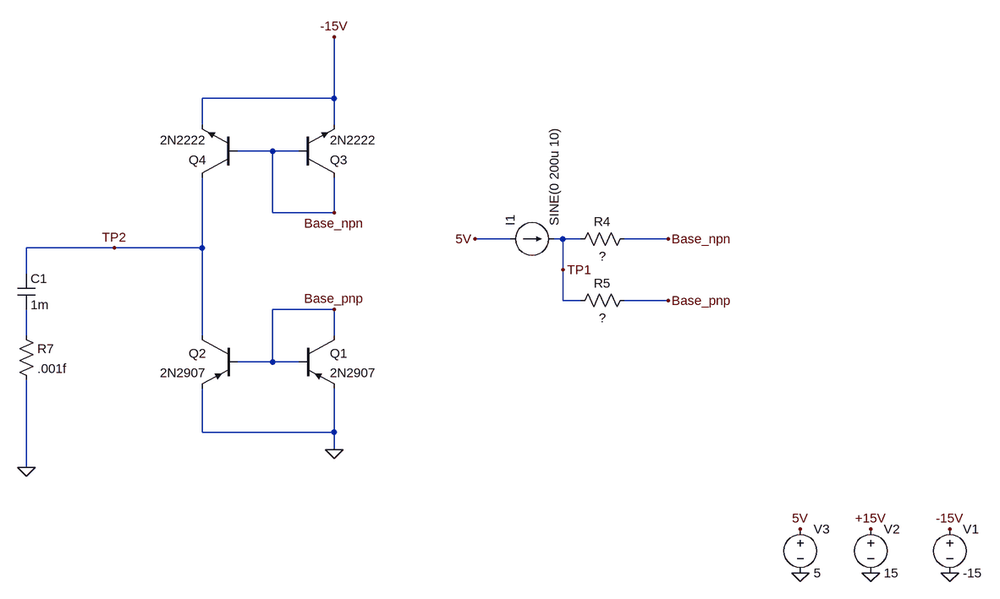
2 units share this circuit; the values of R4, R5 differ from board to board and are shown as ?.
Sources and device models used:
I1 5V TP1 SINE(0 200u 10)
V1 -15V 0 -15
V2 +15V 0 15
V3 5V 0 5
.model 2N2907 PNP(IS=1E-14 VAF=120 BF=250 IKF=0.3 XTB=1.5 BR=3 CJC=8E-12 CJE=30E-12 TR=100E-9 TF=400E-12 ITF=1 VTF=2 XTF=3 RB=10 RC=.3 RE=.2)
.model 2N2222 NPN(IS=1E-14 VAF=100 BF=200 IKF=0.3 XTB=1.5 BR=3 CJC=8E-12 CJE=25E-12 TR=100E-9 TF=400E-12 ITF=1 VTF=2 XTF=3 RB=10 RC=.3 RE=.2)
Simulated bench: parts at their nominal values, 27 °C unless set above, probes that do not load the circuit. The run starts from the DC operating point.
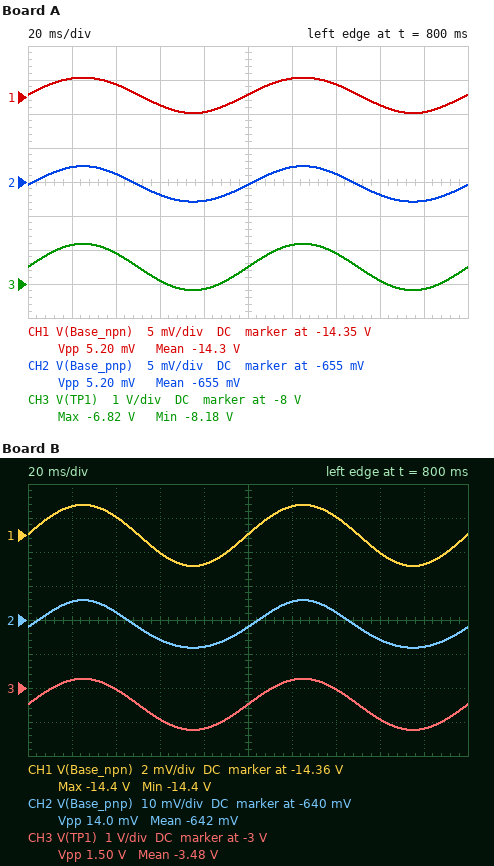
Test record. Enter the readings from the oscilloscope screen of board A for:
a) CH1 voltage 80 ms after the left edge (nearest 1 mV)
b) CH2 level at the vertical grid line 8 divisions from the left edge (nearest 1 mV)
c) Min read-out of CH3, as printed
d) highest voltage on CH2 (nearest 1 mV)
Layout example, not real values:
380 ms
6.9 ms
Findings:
-14.347 V
-657 mV
-8.18 V
-653 mV
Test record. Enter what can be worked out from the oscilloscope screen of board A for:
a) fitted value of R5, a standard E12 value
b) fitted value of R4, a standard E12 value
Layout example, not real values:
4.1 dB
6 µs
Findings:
6.8 kΩ
6.8 kΩ
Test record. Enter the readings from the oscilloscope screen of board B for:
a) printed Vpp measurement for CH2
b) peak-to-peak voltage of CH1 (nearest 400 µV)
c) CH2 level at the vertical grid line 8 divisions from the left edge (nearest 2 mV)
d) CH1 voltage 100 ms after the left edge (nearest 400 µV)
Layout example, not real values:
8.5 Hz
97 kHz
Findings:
14.0 mV
3.6 mV
-646 mV
-14.3580 V
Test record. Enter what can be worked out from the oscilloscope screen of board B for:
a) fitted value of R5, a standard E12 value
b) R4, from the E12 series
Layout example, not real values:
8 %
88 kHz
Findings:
4.7 kΩ
18 kΩ
